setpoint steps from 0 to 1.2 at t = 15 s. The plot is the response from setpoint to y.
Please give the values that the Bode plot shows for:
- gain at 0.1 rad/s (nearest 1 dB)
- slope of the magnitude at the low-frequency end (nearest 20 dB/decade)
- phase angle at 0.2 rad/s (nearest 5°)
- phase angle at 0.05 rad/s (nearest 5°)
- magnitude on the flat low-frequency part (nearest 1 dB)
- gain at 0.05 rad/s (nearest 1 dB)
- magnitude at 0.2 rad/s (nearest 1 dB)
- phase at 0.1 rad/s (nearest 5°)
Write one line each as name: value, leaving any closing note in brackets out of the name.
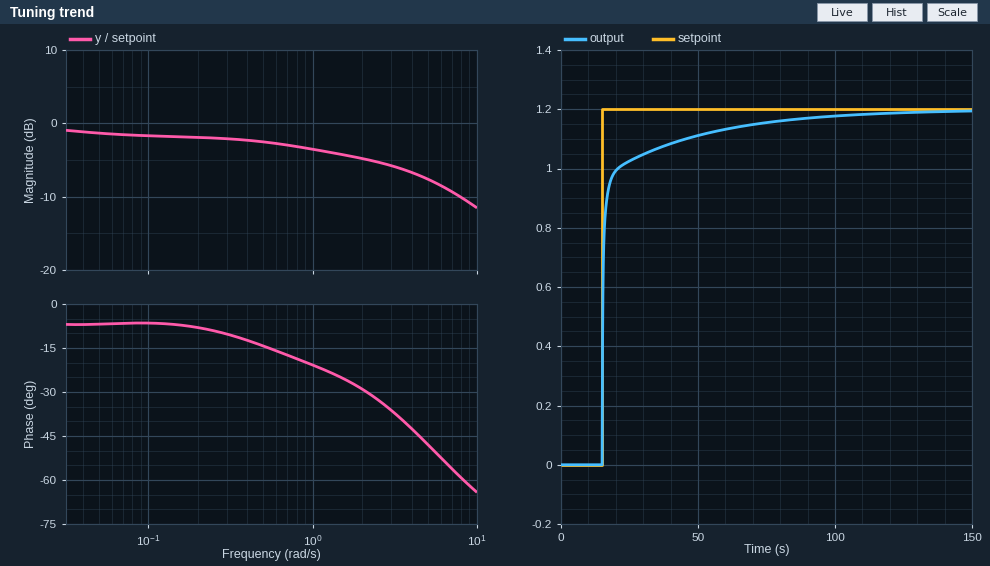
gain at 0.1 rad/s: -2 dB
slope of the magnitude at the low-frequency end: 0 dB/decade
phase angle at 0.2 rad/s: -10°
phase angle at 0.05 rad/s: -5°
magnitude on the flat low-frequency part: -1 dB
gain at 0.05 rad/s: -1 dB
magnitude at 0.2 rad/s: -2 dB
phase at 0.1 rad/s: -5°
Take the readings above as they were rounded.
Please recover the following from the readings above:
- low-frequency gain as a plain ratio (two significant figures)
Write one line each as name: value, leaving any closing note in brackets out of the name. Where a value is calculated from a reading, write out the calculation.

low-frequency gain as a plain ratio: 10^(-1 / 20) = 0.89
